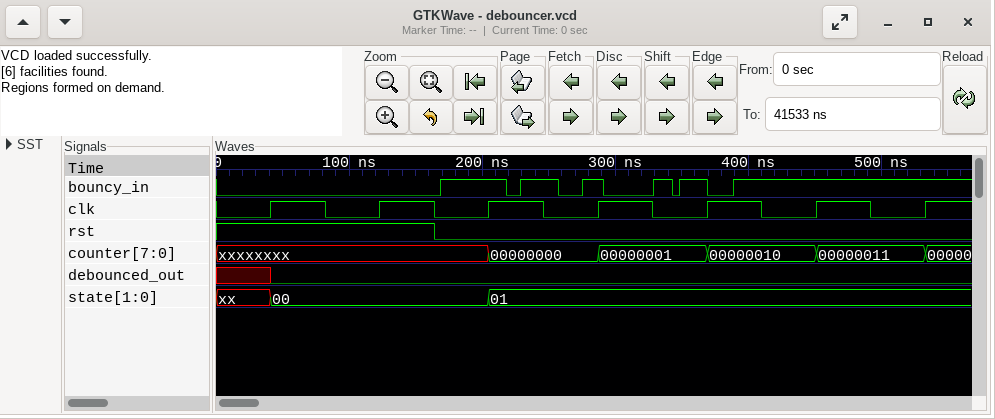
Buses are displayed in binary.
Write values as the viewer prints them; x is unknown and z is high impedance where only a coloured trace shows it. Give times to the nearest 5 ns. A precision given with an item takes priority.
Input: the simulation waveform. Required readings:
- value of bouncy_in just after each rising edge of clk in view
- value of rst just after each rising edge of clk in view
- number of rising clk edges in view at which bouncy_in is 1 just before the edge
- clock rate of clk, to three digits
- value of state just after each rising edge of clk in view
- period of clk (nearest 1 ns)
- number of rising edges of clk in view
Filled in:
0 0 1 1 0 1 1
1 1 0 0 0 0 0
5
12.2 MHz
00, 00, 01, 01, 01, 01, 01
82 ns
7
